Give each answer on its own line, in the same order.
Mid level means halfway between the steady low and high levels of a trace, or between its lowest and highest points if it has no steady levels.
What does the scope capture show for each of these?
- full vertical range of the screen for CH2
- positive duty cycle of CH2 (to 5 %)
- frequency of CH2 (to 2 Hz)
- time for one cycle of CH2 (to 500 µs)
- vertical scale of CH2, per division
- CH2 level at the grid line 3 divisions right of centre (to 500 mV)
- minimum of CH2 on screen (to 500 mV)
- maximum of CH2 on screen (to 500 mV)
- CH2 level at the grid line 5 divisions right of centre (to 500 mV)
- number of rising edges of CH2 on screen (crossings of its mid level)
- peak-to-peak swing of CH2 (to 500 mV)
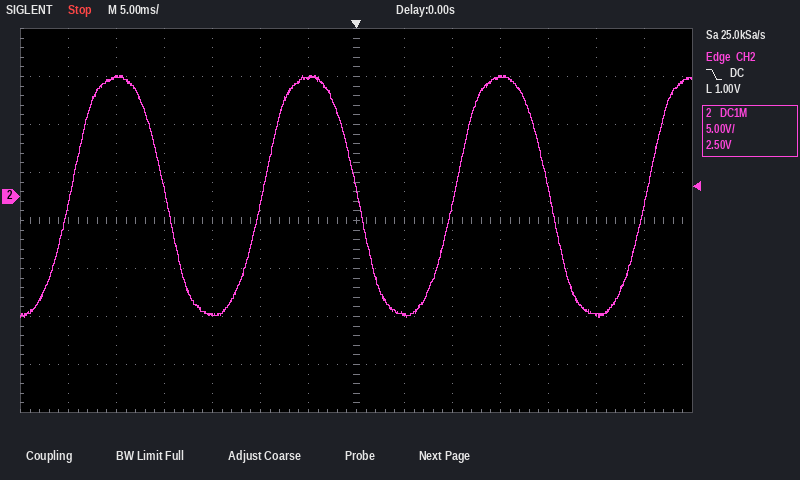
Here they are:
40 V
50 %
50 Hz
20.0 ms
5 V
12.5 V
-12.5 V
12.5 V
-12.5 V
4
25.0 V
